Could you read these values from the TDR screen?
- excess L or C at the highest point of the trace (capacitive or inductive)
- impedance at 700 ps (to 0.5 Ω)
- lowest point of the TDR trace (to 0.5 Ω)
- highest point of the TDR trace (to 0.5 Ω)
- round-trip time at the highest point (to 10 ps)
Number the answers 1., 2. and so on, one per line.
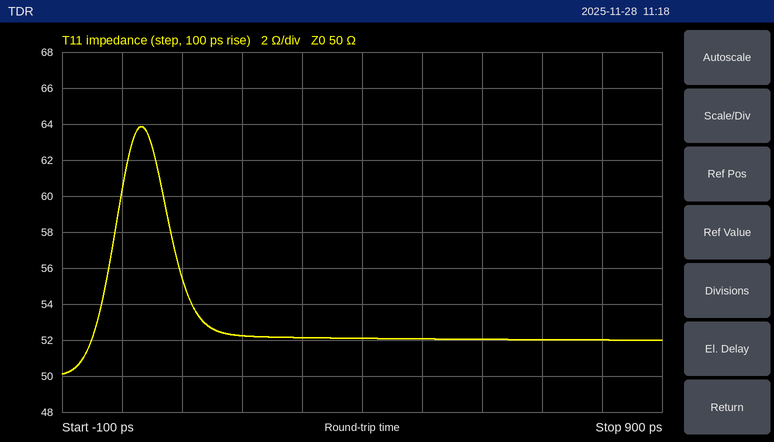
1. inductive
2. 52.0 Ω
3. 50.0 Ω
4. 64.0 Ω
5. 30 ps
